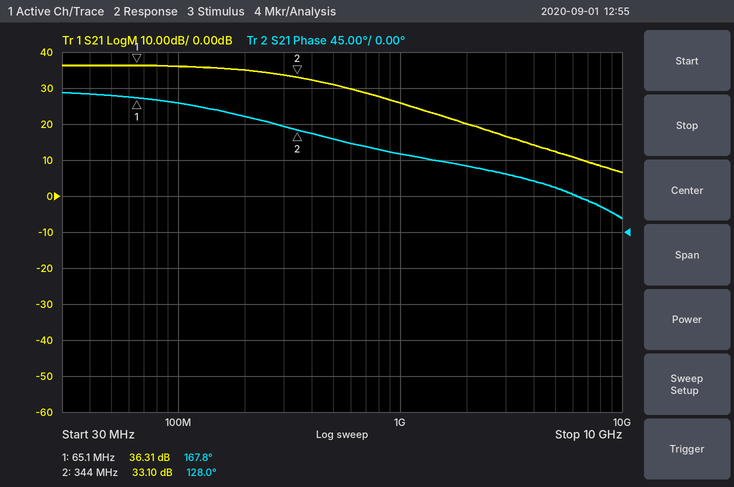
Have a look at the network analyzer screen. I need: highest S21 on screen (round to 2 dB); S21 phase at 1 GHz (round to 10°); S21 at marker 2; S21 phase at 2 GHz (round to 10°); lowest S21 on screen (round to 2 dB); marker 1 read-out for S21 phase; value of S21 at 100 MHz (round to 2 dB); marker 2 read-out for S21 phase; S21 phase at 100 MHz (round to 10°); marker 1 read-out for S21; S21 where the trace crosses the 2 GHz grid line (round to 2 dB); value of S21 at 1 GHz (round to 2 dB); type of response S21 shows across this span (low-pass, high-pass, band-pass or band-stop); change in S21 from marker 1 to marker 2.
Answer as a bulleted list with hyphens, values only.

- 36 dB
- 100°
- 33.10 dB
- 80°
- 6 dB
- 167.8°
- 36 dB
- 128.0°
- 160°
- 36.31 dB
- 20 dB
- 26 dB
- low-pass
- -3.21 dB
